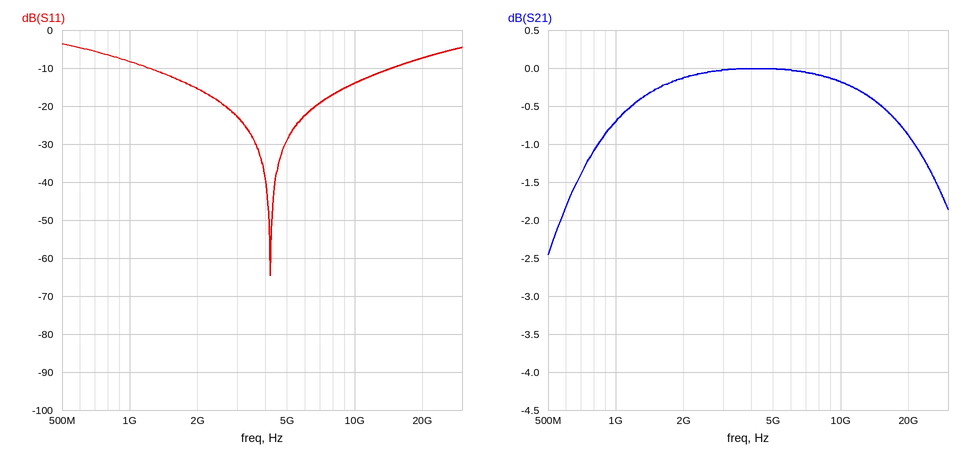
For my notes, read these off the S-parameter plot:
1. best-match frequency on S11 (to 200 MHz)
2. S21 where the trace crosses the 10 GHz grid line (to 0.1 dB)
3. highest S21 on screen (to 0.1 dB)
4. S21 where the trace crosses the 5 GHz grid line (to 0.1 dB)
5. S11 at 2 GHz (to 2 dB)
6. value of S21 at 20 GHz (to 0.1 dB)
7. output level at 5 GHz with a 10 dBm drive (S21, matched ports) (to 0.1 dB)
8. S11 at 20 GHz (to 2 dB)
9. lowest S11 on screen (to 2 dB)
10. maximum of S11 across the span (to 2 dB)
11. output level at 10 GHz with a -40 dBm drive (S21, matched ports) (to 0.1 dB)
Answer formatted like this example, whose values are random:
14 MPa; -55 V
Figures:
4.2 GHz; -0.2 dB; 0.0 dB; 0.0 dB; -16 dB; -0.9 dB; 10.0 dBm; -8 dB; -64 dB; -4 dB; -40.2 dBm
